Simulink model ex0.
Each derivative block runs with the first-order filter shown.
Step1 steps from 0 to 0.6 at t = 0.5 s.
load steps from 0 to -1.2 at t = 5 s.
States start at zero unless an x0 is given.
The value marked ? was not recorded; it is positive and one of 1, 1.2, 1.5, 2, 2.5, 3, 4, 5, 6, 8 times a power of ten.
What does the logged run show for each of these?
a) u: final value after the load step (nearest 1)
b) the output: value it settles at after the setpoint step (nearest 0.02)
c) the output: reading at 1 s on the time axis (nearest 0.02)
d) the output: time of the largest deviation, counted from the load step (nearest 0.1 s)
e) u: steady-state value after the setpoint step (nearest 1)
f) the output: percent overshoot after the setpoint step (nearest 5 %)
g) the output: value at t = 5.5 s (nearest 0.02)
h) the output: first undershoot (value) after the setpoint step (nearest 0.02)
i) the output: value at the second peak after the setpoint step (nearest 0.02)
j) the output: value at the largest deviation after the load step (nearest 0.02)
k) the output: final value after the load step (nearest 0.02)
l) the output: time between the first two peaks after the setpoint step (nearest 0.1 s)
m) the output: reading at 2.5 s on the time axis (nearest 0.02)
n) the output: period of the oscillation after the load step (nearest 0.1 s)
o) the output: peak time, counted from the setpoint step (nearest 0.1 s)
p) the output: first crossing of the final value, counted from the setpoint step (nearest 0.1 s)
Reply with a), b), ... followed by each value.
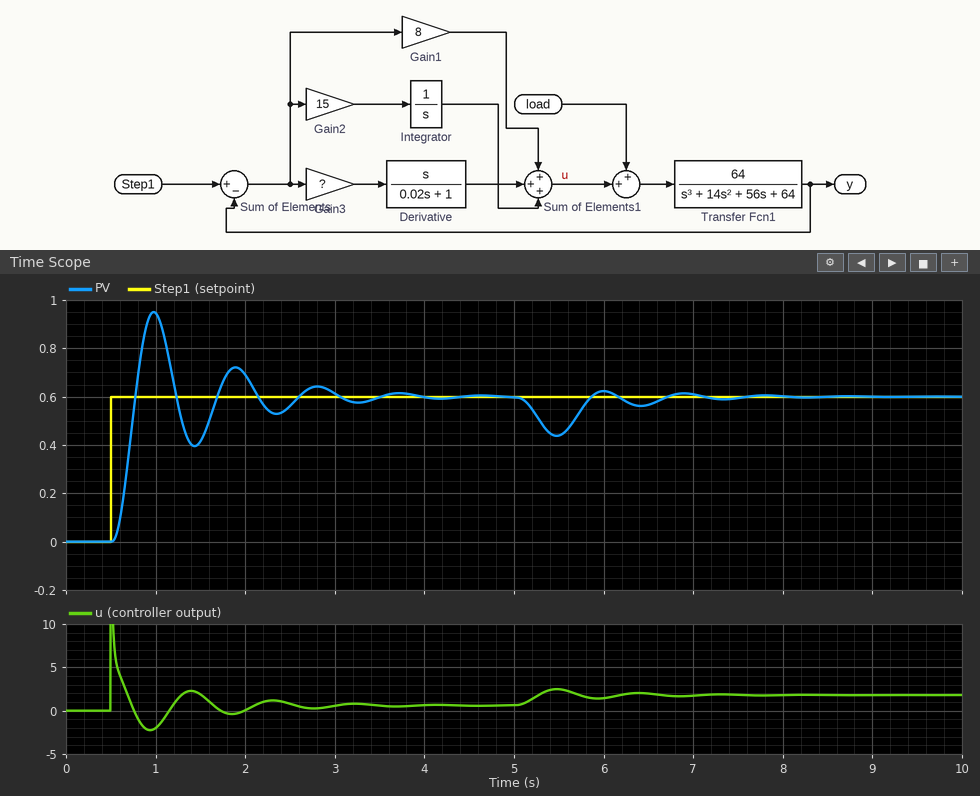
a) 2
b) 0.60
c) 0.94
d) 0.5 s
e) 1
f) 60 %
g) 0.44
h) 0.40
i) 0.72
j) 0.44
k) 0.60
l) 0.9 s
m) 0.56
n) 0.9 s
o) 0.5 s
p) 0.3 s
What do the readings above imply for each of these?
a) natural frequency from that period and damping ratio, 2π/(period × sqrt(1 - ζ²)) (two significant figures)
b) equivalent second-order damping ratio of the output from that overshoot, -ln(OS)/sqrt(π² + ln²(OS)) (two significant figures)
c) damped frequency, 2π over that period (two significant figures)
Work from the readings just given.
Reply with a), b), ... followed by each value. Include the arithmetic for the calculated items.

a) 2π / (0.9 × sqrt(1 - 0.16²)) = 7.1 rad/s
b) ln(0.6) = -0.511; 0.511 / sqrt(9.870 + 0.261) = 0.16
c) 2π / 0.9 = 7.0 rad/s
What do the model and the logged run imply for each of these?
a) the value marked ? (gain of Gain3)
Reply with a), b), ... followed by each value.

a) 0.6
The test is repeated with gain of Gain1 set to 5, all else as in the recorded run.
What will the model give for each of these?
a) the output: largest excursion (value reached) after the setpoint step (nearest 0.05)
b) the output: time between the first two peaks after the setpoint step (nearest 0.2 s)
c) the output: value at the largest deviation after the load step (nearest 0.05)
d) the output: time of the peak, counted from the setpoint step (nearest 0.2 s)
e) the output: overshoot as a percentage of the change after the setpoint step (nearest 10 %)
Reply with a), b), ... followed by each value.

a) 0.90
b) 1.2 s
c) 0.40
d) 0.6 s
e) 50 %
